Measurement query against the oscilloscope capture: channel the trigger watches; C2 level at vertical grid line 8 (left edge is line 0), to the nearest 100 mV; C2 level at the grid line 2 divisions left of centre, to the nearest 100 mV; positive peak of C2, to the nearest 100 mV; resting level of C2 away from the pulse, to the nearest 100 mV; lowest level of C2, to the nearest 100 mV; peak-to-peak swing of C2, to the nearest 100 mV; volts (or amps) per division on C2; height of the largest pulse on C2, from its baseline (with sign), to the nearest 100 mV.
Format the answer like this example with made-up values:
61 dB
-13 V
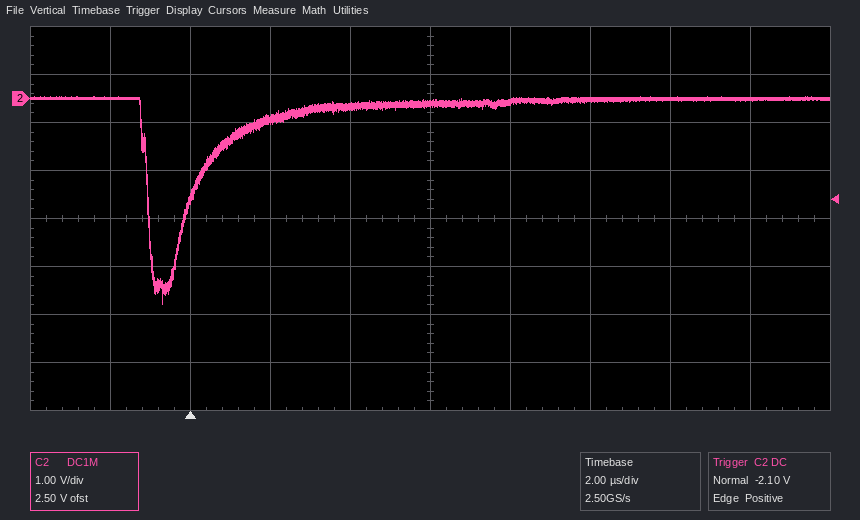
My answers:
C2
0.0 V
-400 mV
0.0 V
0.0 V
-4.3 V
4.3 V
1 V
-4.3 V
